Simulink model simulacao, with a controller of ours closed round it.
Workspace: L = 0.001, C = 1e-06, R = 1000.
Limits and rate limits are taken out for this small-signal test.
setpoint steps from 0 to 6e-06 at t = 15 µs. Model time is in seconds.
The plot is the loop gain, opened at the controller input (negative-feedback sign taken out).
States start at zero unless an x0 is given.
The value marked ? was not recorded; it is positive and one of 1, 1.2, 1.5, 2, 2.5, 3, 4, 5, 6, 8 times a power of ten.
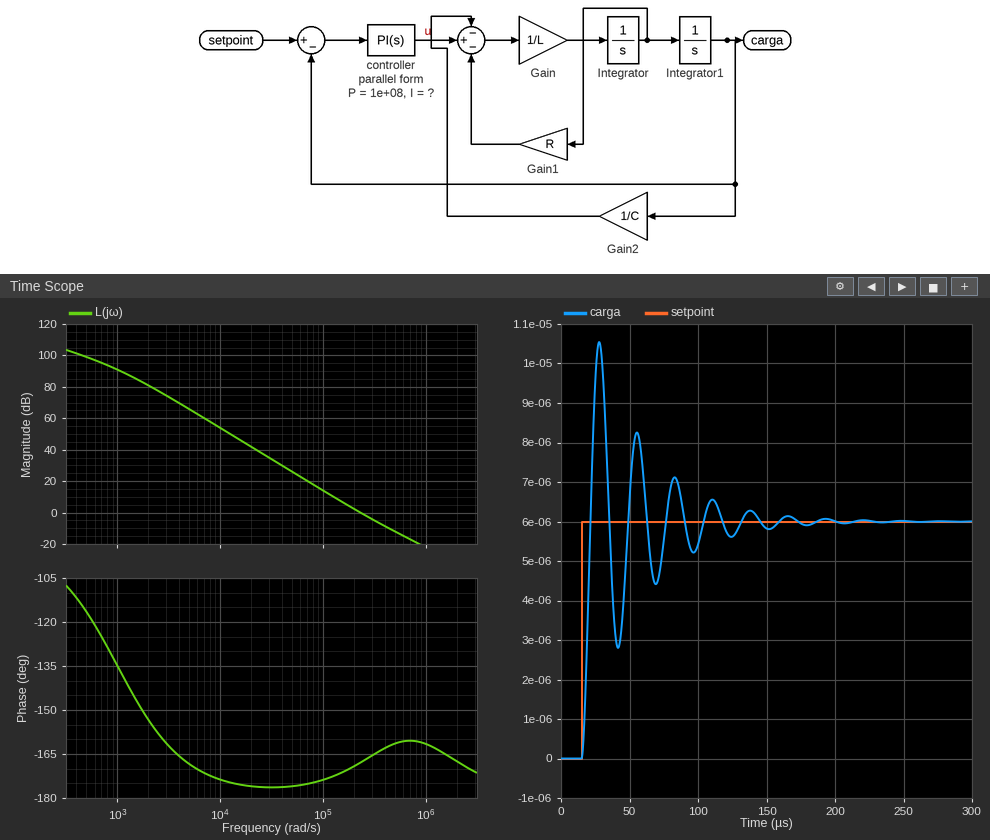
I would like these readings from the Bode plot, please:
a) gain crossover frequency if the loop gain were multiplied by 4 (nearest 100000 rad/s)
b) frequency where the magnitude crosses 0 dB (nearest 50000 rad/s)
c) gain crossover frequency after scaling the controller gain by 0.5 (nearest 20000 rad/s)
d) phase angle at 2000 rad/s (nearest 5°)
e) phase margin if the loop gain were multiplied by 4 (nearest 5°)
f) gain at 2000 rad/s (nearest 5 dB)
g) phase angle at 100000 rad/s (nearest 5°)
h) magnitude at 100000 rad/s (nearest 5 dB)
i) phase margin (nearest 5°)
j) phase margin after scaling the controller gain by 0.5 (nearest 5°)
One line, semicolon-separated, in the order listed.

500000 rad/s; 250000 rad/s; 160000 rad/s; -155°; 20°; 80 dB; -175°; 15 dB; 10°; 10°
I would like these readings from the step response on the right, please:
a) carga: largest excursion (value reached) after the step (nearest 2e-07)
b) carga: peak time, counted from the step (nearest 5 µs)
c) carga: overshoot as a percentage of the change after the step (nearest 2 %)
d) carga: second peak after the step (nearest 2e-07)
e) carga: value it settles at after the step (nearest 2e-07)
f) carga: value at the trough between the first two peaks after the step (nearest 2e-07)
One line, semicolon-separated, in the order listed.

0.0000106; 15 µs; 76 %; 0.0000082; 0.0000060; 0.0000028
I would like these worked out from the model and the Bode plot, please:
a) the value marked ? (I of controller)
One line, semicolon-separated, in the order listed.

5e+13
